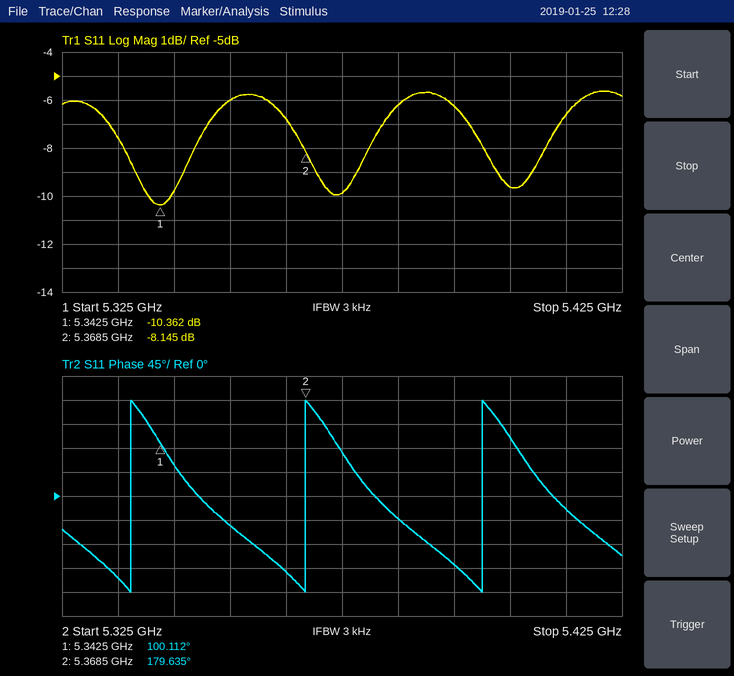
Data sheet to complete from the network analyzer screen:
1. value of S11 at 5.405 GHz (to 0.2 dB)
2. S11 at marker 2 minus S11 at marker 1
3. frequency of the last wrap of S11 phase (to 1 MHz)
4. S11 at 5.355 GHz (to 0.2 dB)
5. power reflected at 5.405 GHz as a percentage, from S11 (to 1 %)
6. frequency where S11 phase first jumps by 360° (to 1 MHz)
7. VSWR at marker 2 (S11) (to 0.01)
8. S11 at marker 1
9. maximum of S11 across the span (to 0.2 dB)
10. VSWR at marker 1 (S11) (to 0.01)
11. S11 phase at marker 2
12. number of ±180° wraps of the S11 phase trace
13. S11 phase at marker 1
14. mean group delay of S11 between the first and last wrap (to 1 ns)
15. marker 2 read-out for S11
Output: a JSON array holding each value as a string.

["-9.6 dB", "2.217 dB", "5.400 GHz", "-6.0 dB", "11 %", "5.337 GHz", "2.29", "-10.362 dB", "-5.6 dB", "1.87", "179.635°", "3", "100.112°", "32 ns", "-8.145 dB"]
